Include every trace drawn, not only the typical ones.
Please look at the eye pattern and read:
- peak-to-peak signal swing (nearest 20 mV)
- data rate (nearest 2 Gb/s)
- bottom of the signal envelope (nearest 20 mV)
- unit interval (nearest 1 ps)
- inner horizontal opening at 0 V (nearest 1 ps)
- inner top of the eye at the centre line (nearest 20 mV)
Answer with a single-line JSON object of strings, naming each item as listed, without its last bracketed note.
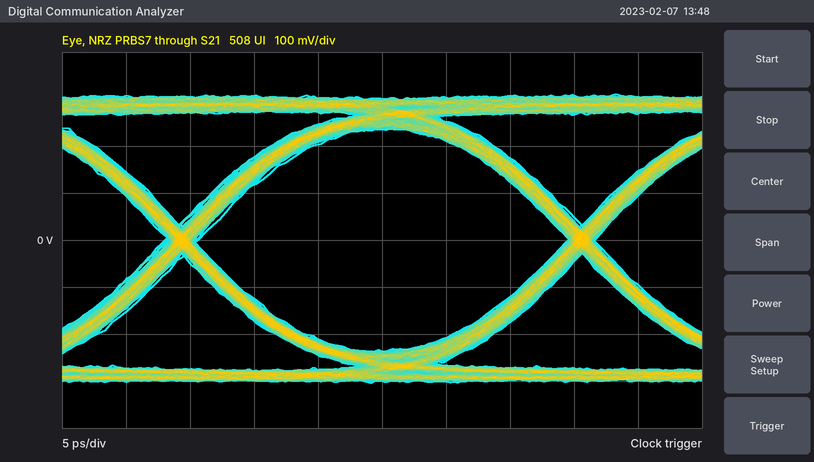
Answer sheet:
{"peak-to-peak signal swing": "620 mV", "data rate": "32 Gb/s", "bottom of the signal envelope": "-300 mV", "unit interval": "31 ps", "inner horizontal opening at 0 V": "29 ps", "inner top of the eye at the centre line": "240 mV"}
